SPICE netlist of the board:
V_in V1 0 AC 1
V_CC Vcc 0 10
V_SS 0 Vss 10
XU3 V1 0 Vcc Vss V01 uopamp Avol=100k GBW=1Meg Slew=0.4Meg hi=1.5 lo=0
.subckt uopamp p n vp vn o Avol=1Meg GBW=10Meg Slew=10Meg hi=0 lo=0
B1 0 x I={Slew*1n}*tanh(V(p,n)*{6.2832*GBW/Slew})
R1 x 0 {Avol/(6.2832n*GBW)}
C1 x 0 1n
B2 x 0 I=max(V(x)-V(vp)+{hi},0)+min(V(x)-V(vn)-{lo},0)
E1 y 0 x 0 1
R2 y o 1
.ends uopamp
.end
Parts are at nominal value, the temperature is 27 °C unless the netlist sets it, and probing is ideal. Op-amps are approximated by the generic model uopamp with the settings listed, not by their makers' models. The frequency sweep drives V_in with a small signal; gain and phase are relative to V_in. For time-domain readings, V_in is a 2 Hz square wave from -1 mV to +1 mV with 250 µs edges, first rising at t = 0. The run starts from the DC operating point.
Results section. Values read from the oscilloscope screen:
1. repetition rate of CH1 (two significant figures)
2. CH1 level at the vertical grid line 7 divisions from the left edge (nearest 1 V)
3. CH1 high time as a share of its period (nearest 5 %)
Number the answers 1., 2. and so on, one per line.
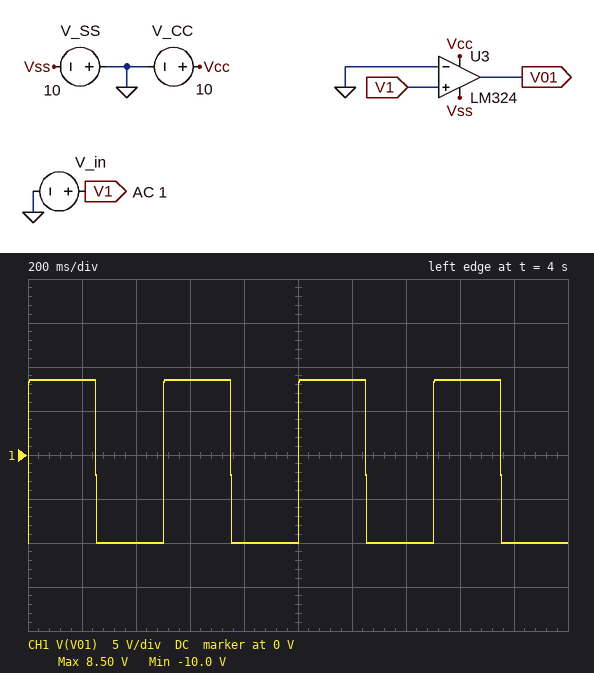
1. 2.0 Hz
2. -10 V
3. 50 %
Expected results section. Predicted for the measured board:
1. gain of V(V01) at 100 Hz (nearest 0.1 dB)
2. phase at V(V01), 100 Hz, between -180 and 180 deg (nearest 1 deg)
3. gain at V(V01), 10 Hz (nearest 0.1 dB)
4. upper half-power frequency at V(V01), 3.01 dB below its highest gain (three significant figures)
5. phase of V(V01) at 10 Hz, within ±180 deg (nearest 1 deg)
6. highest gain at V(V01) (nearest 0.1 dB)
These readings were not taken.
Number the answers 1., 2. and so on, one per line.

1. 80.0 dB
2. -84 deg
3. 97.0 dB
4. 10.0 Hz
5. -45 deg
6. 100.0 dB
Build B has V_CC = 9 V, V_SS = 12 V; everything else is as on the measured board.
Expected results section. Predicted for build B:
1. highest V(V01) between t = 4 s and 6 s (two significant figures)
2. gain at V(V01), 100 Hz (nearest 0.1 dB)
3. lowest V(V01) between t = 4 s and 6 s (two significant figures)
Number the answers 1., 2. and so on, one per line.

1. 7.5 V
2. 80.0 dB
3. -12 V
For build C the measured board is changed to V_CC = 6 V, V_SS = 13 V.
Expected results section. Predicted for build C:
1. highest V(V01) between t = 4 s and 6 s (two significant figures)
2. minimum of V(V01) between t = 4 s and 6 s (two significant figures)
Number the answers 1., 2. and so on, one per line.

1. 4.5 V
2. -13 V
